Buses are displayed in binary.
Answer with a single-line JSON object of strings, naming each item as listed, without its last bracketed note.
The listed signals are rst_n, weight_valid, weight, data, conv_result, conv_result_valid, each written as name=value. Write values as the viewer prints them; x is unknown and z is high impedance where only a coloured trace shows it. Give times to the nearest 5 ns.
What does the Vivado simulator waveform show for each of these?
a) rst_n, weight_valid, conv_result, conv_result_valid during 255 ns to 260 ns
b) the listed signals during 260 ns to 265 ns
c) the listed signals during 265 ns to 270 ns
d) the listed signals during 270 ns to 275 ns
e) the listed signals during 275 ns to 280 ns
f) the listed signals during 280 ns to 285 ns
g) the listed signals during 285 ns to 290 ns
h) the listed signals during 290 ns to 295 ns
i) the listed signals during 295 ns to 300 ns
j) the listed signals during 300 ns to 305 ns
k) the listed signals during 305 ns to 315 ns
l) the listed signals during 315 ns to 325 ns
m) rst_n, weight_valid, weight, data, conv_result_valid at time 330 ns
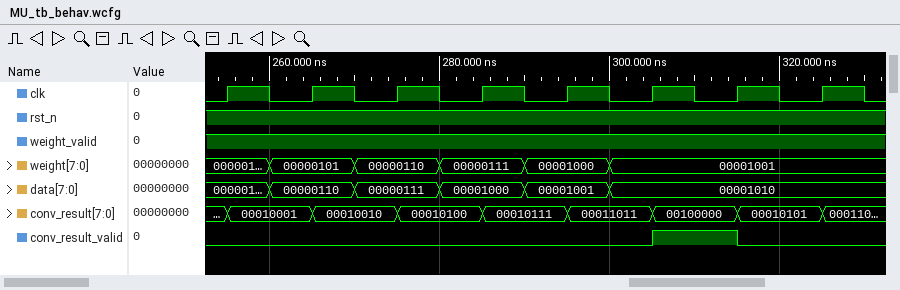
{"rst_n, weight_valid, conv_result, conv_result_valid during 255 ns to 260 ns": "rst_n=1, weight_valid=1, conv_result=00010001, conv_result_valid=0", "the listed signals during 260 ns to 265 ns": "rst_n=1, weight_valid=1, weight=00000101, data=00000110, conv_result=00010001, conv_result_valid=0", "the listed signals during 265 ns to 270 ns": "rst_n=1, weight_valid=1, weight=00000101, data=00000110, conv_result=00010010, conv_result_valid=0", "the listed signals during 270 ns to 275 ns": "rst_n=1, weight_valid=1, weight=00000110, data=00000111, conv_result=00010010, conv_result_valid=0", "the listed signals during 275 ns to 280 ns": "rst_n=1, weight_valid=1, weight=00000110, data=00000111, conv_result=00010100, conv_result_valid=0", "the listed signals during 280 ns to 285 ns": "rst_n=1, weight_valid=1, weight=00000111, data=00001000, conv_result=00010100, conv_result_valid=0", "the listed signals during 285 ns to 290 ns": "rst_n=1, weight_valid=1, weight=00000111, data=00001000, conv_result=00010111, conv_result_valid=0", "the listed signals during 290 ns to 295 ns": "rst_n=1, weight_valid=1, weight=00001000, data=00001001, conv_result=00010111, conv_result_valid=0", "the listed signals during 295 ns to 300 ns": "rst_n=1, weight_valid=1, weight=00001000, data=00001001, conv_result=00011011, conv_result_valid=0", "the listed signals during 300 ns to 305 ns": "rst_n=1, weight_valid=1, weight=00001001, data=00001010, conv_result=00011011, conv_result_valid=0", "the listed signals during 305 ns to 315 ns": "rst_n=1, weight_valid=1, weight=00001001, data=00001010, conv_result=00100000, conv_result_valid=1", "the listed signals during 315 ns to 325 ns": "rst_n=1, weight_valid=1, weight=00001001, data=00001010, conv_result=00010101, conv_result_valid=0", "rst_n, weight_valid, weight, data, conv_result_valid at time 330 ns": "rst_n=1, weight_valid=1, weight=00001001, data=00001010, conv_result_valid=0"}
